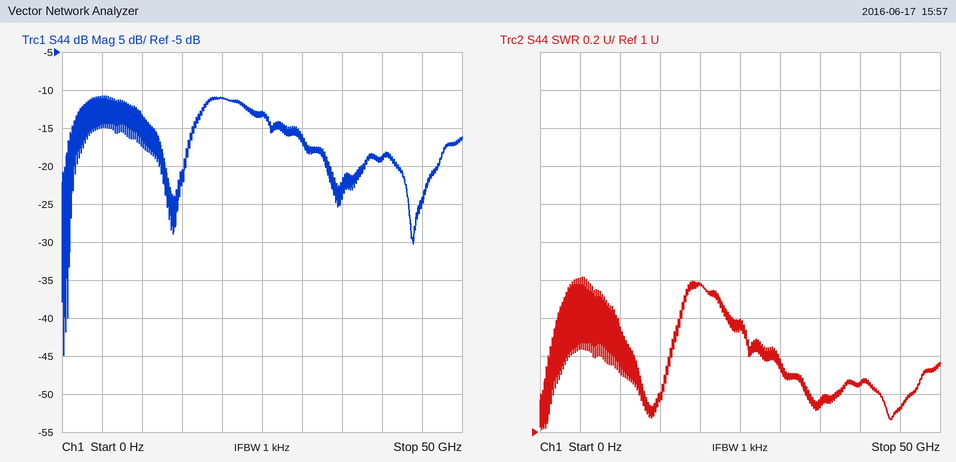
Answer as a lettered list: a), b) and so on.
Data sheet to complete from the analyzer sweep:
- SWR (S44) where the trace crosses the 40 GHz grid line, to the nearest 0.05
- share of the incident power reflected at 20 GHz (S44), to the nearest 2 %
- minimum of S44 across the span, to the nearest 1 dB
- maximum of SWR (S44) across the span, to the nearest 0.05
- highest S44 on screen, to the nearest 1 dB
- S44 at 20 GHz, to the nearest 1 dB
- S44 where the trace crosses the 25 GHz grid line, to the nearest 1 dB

a) 1.25
b) 8 %
c) -45 dB
d) 1.80
e) -11 dB
f) -11 dB
g) -13 dB
